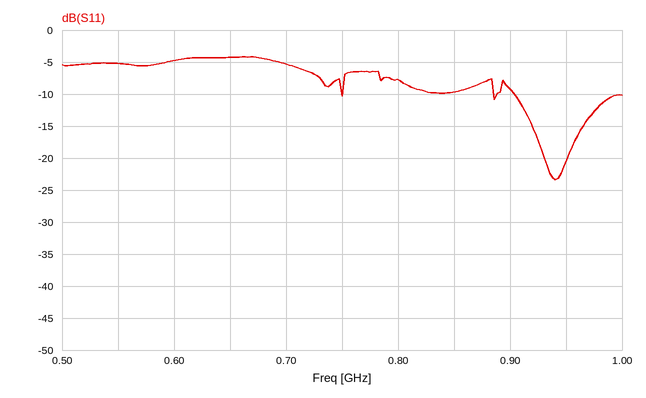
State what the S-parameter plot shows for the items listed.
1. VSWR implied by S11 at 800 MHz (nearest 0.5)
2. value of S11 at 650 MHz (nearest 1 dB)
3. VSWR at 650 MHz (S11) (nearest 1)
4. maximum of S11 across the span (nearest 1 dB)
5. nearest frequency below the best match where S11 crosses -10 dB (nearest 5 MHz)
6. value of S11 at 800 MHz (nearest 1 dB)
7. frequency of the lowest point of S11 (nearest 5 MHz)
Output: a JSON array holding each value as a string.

["2.5", "-4 dB", "4", "-4 dB", "905 MHz", "-8 dB", "940 MHz"]
